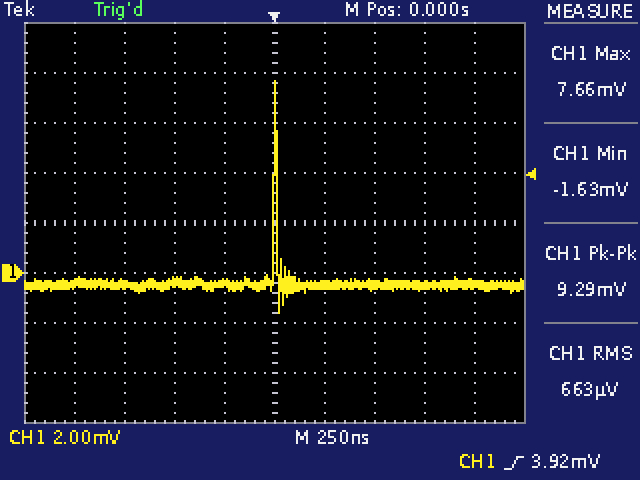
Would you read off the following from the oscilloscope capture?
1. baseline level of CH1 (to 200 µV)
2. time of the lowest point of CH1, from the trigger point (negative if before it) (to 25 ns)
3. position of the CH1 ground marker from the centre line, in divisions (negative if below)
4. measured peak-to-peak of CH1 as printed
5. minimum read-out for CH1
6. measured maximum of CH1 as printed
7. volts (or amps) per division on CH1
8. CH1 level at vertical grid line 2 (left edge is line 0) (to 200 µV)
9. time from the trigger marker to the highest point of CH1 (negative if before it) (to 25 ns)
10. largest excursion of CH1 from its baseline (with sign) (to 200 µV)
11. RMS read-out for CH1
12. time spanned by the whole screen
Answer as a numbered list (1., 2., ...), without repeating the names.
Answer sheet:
1. -400 µV
2. +25 ns
3. -1.0 div
4. 9.29 mV
5. -1.63 mV
6. 7.66 mV
7. 2 mV
8. -400 µV
9. 0 ns
10. +8.2 mV
11. 663 µV
12. 2.5 µs
